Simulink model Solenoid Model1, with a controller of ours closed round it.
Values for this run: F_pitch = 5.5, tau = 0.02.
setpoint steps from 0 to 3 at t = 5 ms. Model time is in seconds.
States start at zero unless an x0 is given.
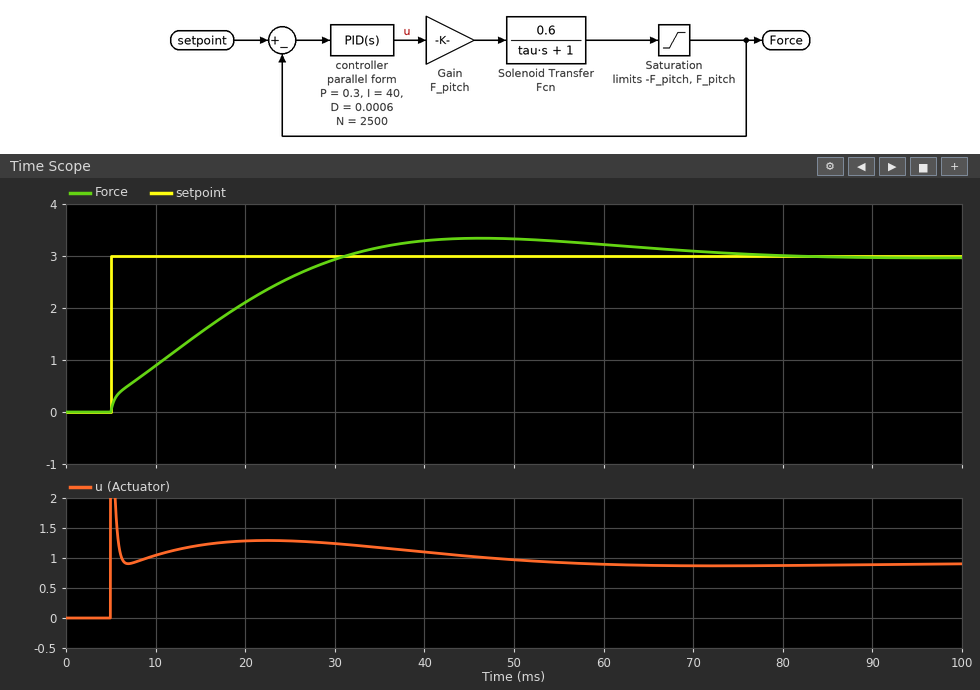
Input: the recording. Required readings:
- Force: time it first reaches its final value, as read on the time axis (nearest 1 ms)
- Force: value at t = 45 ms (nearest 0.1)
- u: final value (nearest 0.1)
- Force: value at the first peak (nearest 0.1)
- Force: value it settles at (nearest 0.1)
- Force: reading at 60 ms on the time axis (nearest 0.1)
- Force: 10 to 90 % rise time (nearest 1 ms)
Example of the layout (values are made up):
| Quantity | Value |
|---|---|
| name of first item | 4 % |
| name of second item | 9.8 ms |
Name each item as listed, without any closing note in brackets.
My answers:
| Quantity | Value |
|---|---|
| Force: time it first reaches its final value, as read on the time axis | 31 ms |
| Force: value at t = 45 ms | 3.3 |
| u: final value | 0.9 |
| Force: value at the first peak | 3.3 |
| Force: value it settles at | 3.0 |
| Force: reading at 60 ms on the time axis | 3.2 |
| Force: 10 to 90 % rise time | 21 ms |
